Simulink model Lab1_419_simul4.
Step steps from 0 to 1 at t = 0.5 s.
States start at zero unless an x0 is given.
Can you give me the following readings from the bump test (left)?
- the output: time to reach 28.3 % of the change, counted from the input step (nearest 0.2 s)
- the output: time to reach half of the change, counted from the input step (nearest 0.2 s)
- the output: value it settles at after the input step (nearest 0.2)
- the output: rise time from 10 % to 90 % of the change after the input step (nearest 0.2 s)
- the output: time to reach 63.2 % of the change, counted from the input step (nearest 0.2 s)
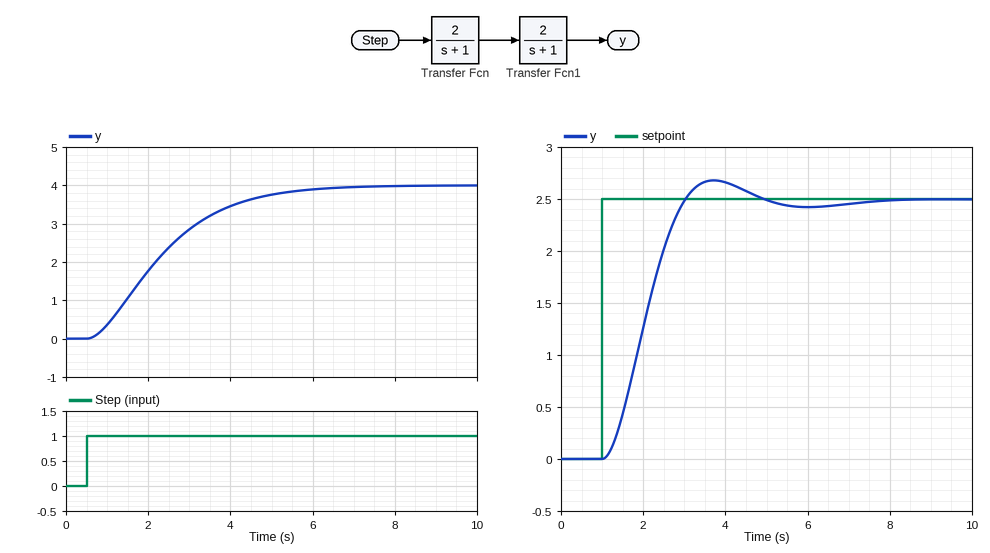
1.0 s
1.6 s
4.0
3.4 s
2.2 s
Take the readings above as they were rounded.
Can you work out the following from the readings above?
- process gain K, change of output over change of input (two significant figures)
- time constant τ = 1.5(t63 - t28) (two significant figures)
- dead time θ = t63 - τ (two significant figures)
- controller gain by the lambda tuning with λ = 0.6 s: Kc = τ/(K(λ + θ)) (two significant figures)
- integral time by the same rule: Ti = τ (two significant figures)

4.0
1.8 s
0.40 s
0.45
1.8 s
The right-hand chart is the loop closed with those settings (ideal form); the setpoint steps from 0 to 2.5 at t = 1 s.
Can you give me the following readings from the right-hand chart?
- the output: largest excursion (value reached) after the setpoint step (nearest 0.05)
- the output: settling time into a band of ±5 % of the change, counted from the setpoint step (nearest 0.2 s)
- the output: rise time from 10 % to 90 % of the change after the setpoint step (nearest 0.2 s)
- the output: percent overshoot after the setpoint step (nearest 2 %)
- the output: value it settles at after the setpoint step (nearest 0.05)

2.70
3.2 s
1.4 s
8 %
2.50
